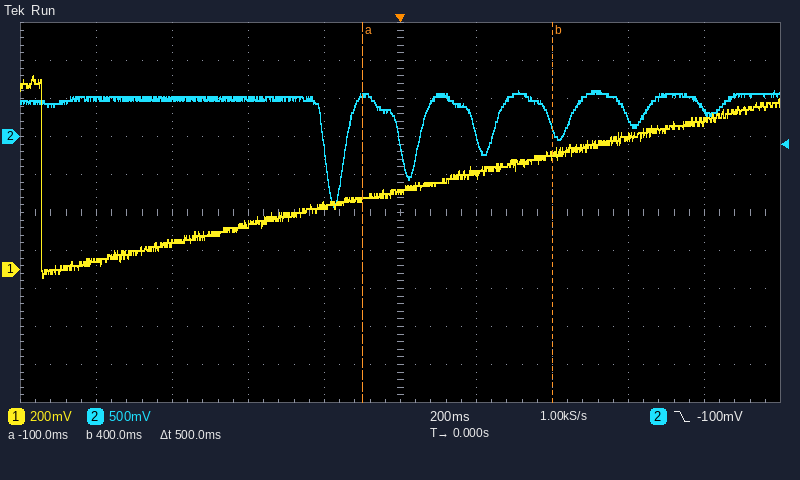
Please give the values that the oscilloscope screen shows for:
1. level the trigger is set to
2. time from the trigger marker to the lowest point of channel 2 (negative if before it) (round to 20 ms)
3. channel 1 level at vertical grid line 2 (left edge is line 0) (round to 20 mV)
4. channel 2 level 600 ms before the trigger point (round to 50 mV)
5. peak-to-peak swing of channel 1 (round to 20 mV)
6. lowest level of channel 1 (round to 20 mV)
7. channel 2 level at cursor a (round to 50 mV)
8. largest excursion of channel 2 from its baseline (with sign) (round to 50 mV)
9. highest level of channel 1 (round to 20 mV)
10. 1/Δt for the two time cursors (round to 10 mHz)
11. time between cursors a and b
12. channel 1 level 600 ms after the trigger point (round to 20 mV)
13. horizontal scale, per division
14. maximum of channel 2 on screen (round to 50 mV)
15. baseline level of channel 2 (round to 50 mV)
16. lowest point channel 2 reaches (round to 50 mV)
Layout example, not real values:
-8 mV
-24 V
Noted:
-100 mV
-180 ms
140 mV
500 mV
1.06 V
-40 mV
550 mV
-1.40 V
1.02 V
2.00 Hz
500 ms
700 mV
200 ms
600 mV
500 mV
-900 mV
